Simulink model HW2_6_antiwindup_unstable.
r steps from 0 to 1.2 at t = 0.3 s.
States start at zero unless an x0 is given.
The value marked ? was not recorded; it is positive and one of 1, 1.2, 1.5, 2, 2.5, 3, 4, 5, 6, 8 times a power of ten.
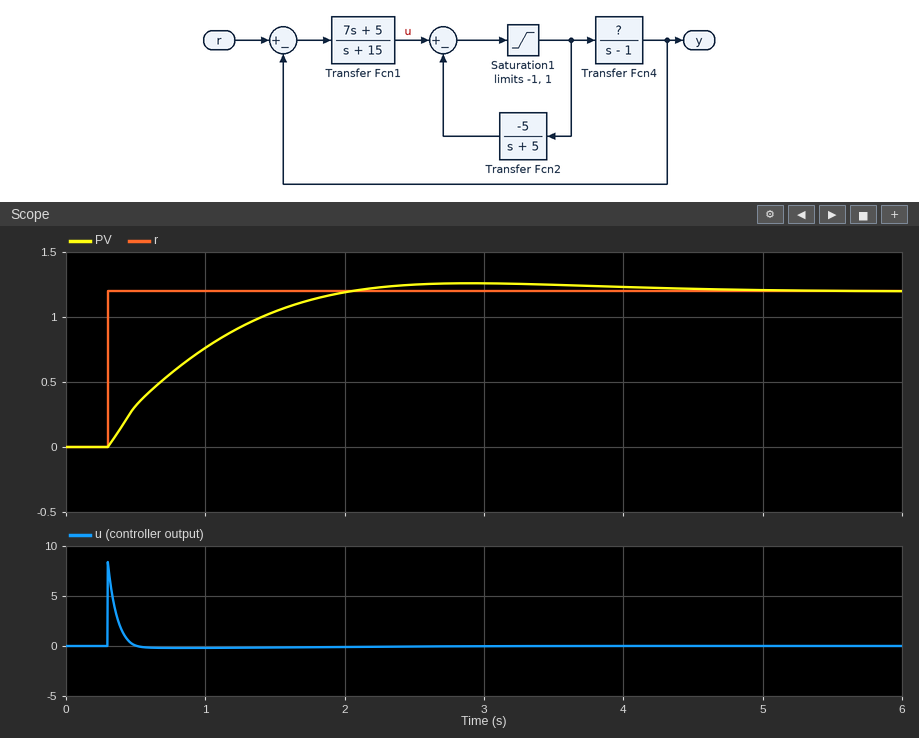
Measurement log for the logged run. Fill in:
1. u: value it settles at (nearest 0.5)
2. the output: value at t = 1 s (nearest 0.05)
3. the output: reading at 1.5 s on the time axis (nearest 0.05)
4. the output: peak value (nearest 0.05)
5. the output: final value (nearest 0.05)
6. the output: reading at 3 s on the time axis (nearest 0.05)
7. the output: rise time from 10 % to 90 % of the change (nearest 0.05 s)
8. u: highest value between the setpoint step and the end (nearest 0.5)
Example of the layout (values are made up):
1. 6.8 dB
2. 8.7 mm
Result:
1. 0.0
2. 0.75
3. 1.05
4. 1.25
5. 1.20
6. 1.25
7. 1.20 s
8. 8.5
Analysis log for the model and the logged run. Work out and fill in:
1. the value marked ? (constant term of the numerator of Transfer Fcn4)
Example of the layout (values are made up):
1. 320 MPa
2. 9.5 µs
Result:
1. 1.5
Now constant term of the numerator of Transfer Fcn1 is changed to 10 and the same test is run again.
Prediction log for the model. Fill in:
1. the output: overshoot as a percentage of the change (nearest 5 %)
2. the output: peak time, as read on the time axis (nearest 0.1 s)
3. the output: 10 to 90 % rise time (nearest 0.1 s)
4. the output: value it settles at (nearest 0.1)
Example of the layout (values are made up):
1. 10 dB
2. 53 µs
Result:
1. 10 %
2. 2.0 s
3. 0.8 s
4. 1.2
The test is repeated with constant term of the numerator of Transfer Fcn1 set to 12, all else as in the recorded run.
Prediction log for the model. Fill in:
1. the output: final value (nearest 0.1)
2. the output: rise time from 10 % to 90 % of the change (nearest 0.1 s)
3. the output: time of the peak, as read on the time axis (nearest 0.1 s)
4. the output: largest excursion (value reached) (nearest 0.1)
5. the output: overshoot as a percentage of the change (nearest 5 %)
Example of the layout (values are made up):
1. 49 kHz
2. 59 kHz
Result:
1. 1.2
2. 0.7 s
3. 1.8 s
4. 1.4
5. 15 %
